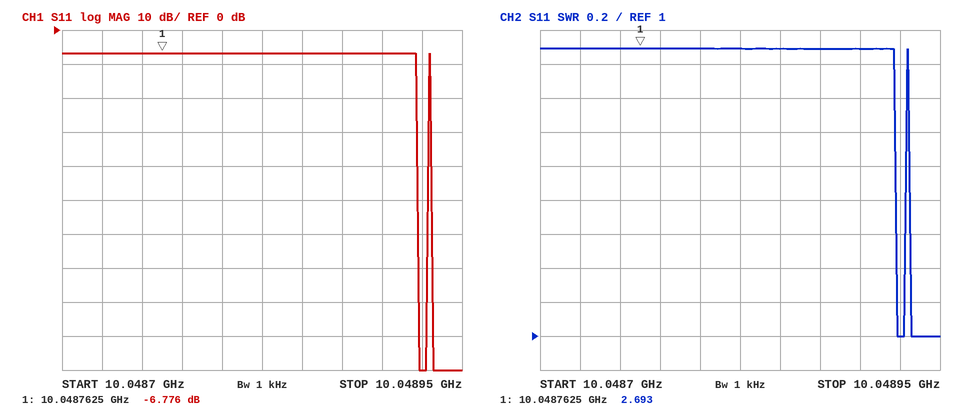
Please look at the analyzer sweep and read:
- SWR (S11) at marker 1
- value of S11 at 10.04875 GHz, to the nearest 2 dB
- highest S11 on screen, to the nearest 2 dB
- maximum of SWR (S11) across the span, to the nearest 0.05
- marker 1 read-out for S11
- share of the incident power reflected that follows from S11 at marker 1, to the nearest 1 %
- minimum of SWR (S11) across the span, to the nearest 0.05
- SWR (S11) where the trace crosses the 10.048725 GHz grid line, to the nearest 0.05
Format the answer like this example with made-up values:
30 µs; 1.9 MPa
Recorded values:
2.693; -6 dB; -6 dB; 2.70; -6.776 dB; 21 %; 1.00; 2.70
